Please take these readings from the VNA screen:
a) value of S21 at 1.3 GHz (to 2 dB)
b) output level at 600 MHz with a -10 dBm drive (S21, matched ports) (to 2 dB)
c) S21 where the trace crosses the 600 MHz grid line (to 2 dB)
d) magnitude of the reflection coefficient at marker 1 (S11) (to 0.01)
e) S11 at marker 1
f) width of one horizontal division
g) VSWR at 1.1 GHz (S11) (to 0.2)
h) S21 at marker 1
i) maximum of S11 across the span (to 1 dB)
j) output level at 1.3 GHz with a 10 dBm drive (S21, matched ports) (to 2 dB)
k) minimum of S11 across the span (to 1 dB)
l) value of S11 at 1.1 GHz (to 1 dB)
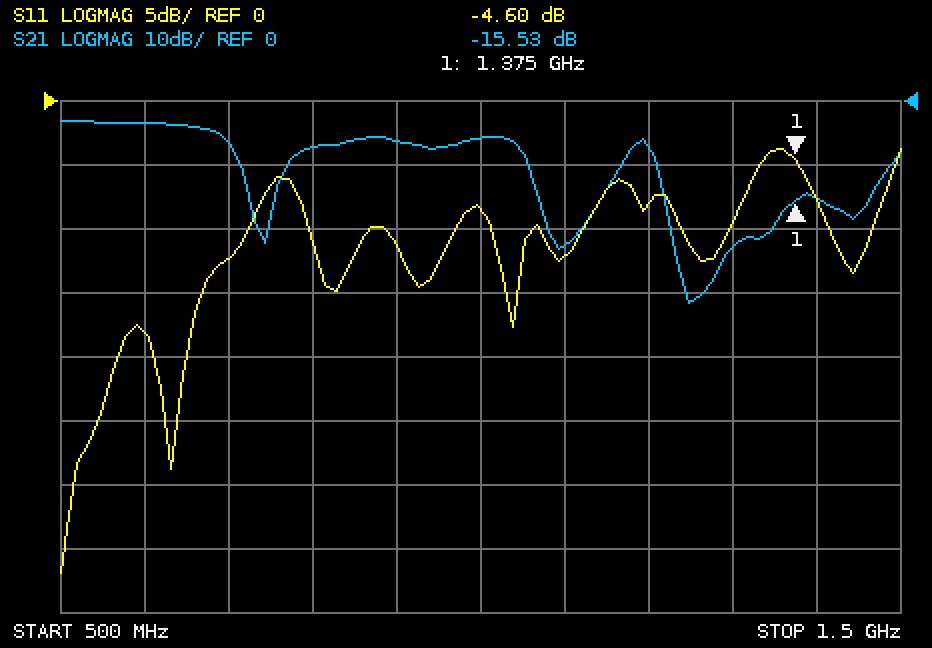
-22 dB
-14 dBm
-4 dB
0.59
-4.60 dB
100 MHz
1.6
-15.53 dB
-4 dB
-12 dBm
-37 dB
-12 dB
